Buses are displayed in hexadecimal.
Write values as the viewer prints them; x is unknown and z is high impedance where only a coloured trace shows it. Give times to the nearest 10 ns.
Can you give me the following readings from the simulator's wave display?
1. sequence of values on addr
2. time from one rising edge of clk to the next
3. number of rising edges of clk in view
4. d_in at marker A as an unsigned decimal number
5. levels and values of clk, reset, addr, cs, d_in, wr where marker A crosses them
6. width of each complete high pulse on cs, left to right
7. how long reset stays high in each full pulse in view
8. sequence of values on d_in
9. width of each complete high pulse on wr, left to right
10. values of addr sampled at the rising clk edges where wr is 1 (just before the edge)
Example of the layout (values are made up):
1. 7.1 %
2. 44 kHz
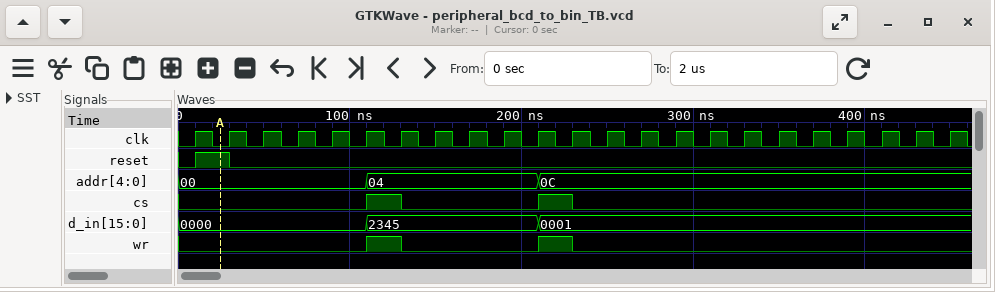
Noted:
1. 00, 04, 0C
2. 20 ns
3. 23
4. 0
5. clk=0, reset=1, addr=00, cs=0, d_in=0000, wr=0
6. 20 ns, 20 ns
7. 20 ns
8. 0000, 2345, 0001
9. 20 ns, 20 ns
10. 04, 0C
